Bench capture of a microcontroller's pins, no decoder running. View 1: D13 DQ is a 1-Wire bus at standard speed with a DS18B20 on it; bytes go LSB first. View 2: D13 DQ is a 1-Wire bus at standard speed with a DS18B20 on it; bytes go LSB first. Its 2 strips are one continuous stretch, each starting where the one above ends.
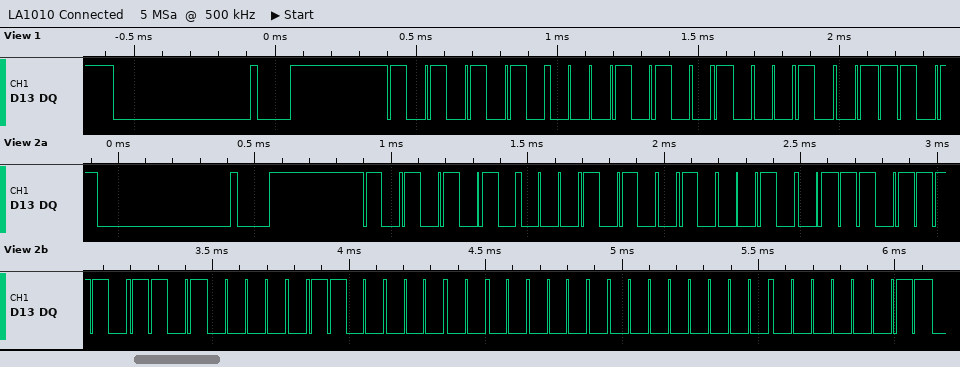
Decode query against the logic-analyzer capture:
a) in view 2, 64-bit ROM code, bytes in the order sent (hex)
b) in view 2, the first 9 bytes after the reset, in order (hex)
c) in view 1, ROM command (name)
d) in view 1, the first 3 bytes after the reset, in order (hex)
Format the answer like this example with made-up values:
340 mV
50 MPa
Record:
28 91 7B 0B 06 00 00 C0
55 28 91 7B 0B 06 00 00 C0
Match ROM
55 28 91
